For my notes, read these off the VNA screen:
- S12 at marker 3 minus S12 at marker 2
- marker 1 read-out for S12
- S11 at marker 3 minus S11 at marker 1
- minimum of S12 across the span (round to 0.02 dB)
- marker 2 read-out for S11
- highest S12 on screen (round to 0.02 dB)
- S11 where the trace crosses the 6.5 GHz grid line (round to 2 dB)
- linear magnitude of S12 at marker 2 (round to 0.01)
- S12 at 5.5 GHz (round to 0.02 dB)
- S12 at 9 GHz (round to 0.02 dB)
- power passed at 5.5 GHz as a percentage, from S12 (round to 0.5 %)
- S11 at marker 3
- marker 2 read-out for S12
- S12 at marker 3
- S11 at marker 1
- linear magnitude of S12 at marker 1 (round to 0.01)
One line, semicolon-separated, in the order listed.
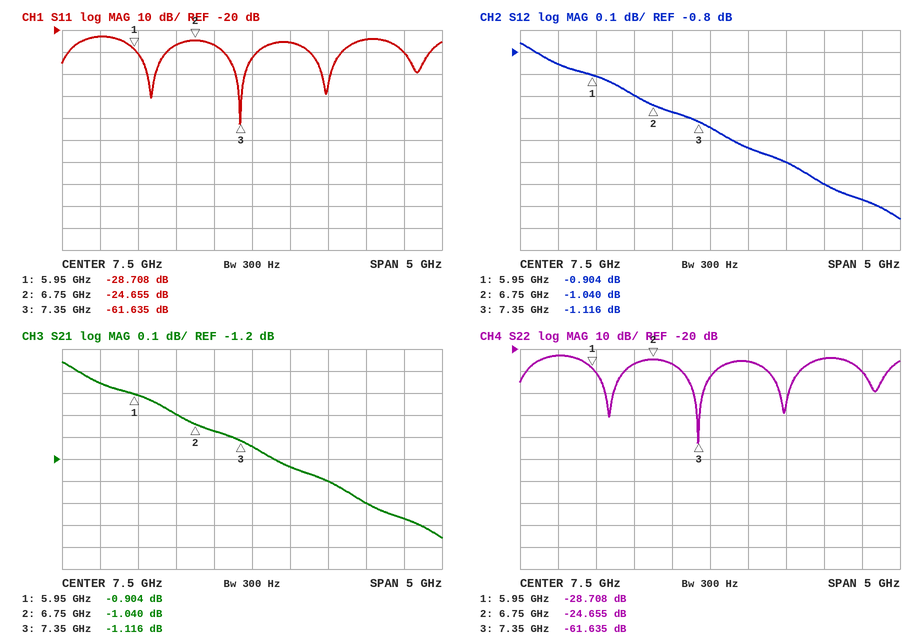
-0.076 dB; -0.904 dB; -32.927 dB; -1.56 dB; -24.655 dB; -0.76 dB; -26 dB; 0.89; -0.86 dB; -1.40 dB; 82.0 %; -61.635 dB; -1.040 dB; -1.116 dB; -28.708 dB; 0.90
